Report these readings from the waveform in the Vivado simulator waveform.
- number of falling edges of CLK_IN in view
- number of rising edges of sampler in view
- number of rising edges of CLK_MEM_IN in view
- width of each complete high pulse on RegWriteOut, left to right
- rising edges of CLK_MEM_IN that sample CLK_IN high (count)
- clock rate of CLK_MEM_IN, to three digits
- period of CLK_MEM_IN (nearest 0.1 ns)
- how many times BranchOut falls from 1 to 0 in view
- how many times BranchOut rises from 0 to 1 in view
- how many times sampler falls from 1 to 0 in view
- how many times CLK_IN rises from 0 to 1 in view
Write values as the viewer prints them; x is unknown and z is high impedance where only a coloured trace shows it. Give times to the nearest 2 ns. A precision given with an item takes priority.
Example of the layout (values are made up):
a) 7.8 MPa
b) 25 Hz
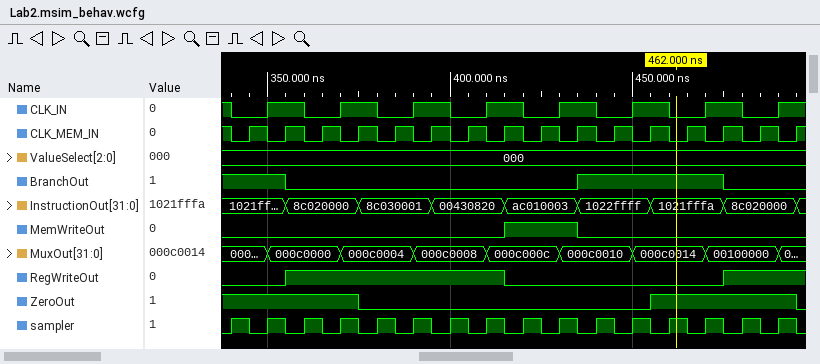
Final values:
a) 8
b) 16
c) 16
d) 60 ns
e) 8
f) 100 MHz
g) 10 ns
h) 2
i) 1
j) 16
k) 8
